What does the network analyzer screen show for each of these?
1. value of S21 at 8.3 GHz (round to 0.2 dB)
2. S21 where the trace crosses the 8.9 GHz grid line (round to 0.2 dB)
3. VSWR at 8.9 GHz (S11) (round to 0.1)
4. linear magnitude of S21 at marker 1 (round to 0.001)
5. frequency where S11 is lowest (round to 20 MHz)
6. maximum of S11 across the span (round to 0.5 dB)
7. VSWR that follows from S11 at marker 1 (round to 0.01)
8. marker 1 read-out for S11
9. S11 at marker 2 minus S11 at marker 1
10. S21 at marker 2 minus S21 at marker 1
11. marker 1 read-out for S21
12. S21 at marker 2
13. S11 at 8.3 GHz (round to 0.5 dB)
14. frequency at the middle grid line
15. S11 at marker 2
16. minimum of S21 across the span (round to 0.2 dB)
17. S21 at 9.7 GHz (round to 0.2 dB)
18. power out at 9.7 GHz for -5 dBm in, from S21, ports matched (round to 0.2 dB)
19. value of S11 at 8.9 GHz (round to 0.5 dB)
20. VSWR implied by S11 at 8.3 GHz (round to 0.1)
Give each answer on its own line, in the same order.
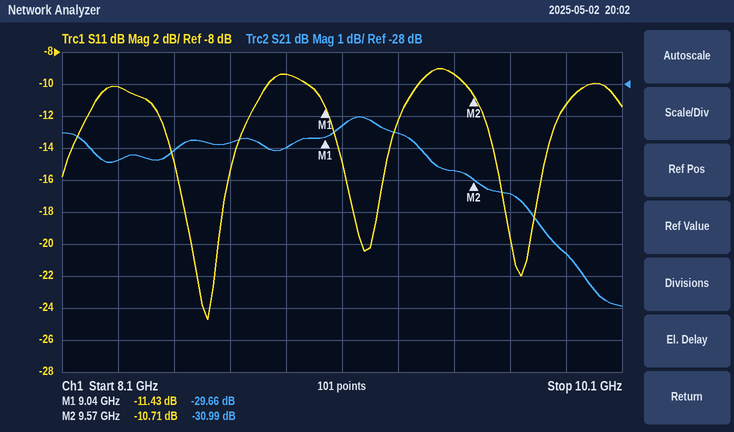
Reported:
-30.4 dB
-30.0 dB
2.0
0.033
8.62 GHz
-9.0 dB
1.73
-11.43 dB
0.72 dB
-1.33 dB
-29.66 dB
-30.99 dB
-10.0 dB
9.1 GHz
-10.71 dB
-35.0 dB
-31.4 dB
-36.4 dBm
-9.5 dB
1.9
